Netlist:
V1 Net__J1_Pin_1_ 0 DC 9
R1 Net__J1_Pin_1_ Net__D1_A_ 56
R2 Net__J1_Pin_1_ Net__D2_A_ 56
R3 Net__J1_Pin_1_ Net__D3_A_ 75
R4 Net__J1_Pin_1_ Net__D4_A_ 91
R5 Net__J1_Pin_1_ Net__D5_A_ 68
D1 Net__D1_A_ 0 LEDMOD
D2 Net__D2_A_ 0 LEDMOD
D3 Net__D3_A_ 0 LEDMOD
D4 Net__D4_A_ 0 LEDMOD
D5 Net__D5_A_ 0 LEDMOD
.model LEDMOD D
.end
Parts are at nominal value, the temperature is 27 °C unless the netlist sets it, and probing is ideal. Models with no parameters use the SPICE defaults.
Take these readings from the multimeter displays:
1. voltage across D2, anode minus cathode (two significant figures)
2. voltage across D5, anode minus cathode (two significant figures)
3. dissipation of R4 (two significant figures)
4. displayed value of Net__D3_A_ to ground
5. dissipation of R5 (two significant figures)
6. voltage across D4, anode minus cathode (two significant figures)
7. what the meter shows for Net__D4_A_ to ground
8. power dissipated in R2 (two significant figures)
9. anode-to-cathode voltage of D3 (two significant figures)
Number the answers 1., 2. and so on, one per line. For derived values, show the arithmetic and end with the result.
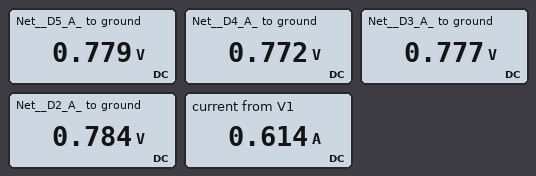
1. 784 mV = 780 mV
2. 779 mV = 780 mV
3. (9 V - 772 mV)^2 / 91 Ω = 740 mW
4. 0.777 V
5. (9 V - 779 mV)^2 / 68 Ω = 990 mW
6. 772 mV = 770 mV
7. 0.772 V
8. (9 V - 784 mV)^2 / 56 Ω = 1.2 W
9. 777 mV = 780 mV
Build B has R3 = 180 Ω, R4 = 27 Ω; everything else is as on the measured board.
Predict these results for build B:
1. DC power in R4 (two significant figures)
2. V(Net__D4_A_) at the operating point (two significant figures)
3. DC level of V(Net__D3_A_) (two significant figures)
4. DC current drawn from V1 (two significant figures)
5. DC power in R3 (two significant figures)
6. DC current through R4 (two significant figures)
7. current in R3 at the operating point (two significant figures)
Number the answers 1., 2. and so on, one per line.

1. 2.5 W
2. 800 mV
3. 750 mV
4. 760 mA
5. 380 mW
6. 300 mA
7. 46 mA
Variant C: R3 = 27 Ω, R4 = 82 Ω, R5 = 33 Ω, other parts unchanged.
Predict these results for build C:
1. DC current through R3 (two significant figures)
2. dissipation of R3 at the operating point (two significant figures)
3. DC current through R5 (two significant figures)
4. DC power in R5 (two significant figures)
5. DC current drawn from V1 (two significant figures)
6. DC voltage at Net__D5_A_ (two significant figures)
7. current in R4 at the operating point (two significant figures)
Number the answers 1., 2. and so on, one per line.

1. 300 mA
2. 2.5 W
3. 250 mA
4. 2.0 W
5. 950 mA
6. 800 mV
7. 100 mA
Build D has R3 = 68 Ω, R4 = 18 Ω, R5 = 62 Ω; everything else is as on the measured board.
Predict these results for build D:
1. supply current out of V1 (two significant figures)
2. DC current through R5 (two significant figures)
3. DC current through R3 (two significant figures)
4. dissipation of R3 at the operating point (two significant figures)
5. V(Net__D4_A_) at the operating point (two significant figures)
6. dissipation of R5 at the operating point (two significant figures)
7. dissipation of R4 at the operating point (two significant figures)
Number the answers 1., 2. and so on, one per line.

1. 1.0 A
2. 130 mA
3. 120 mA
4. 990 mW
5. 810 mV
6. 1.1 W
7. 3.7 W
